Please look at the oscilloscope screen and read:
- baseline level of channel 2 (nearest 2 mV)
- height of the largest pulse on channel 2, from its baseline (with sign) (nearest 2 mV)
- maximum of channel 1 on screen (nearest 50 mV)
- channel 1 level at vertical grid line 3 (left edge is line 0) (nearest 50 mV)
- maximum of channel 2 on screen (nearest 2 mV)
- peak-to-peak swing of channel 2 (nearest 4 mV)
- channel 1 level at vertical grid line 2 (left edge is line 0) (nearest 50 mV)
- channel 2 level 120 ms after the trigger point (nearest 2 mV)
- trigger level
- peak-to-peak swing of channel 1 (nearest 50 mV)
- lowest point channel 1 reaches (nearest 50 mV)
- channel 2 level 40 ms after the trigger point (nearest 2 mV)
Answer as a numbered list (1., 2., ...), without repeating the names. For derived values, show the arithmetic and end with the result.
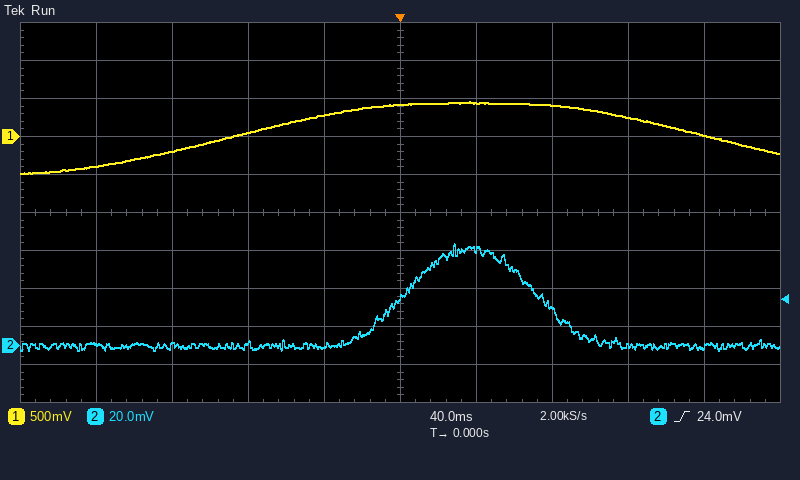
1. 0 mV
2. 54 mV − (0 mV) = +54 mV
3. 450 mV
4. 50 mV
5. 54 mV
6. 56 mV
7. -200 mV
8. 0 mV
9. 24.0 mV
10. 450 mV − (-500 mV) = 950 mV
11. -500 mV
12. 50 mV
